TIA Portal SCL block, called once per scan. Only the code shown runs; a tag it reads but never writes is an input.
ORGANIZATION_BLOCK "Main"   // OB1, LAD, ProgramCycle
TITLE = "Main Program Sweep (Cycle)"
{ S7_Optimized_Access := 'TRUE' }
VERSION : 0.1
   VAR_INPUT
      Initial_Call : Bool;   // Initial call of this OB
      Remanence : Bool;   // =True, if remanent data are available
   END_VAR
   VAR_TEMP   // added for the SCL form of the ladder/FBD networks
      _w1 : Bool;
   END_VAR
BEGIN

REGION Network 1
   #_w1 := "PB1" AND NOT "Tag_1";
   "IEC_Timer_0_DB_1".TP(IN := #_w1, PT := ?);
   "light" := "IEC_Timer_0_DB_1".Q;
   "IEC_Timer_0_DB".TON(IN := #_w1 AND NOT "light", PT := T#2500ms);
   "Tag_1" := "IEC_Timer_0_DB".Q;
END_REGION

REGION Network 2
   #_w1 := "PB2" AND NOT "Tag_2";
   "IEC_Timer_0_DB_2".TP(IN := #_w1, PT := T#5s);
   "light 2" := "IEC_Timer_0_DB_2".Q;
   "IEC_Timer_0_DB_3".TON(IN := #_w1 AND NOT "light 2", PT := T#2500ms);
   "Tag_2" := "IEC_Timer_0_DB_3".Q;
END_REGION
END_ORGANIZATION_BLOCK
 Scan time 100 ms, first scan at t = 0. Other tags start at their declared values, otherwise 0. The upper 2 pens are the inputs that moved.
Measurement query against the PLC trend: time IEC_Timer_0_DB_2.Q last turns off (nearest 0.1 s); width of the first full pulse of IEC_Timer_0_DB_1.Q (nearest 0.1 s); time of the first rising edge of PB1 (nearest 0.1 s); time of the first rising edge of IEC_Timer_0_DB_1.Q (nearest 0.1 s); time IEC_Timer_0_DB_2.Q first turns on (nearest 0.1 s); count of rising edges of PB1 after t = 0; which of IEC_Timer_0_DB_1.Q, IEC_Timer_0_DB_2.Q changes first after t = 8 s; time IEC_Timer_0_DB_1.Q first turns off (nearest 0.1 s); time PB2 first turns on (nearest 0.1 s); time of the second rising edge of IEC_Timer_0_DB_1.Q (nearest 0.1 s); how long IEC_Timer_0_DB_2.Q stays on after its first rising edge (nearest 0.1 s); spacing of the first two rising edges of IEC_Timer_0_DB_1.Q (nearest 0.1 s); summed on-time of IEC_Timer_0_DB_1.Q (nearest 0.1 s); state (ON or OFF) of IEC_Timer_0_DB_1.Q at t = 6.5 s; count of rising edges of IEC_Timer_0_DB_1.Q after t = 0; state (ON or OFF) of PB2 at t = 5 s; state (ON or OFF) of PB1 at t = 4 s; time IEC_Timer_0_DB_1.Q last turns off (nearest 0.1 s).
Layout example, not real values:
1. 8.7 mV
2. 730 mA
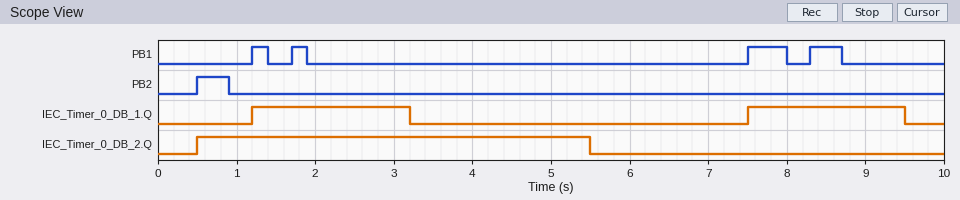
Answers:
1. 5.5 s
2. 2.0 s
3. 1.2 s
4. 1.2 s
5. 0.5 s
6. 4
7. IEC_Timer_0_DB_1.Q
8. 3.2 s
9. 0.5 s
10. 7.5 s
11. 5.0 s
12. 6.3 s
13. 4.0 s
14. OFF
15. 2
16. OFF
17. OFF
18. 9.5 s
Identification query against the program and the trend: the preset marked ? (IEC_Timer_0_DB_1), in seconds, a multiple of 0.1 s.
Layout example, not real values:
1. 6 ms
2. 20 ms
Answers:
1. 2.0 s
